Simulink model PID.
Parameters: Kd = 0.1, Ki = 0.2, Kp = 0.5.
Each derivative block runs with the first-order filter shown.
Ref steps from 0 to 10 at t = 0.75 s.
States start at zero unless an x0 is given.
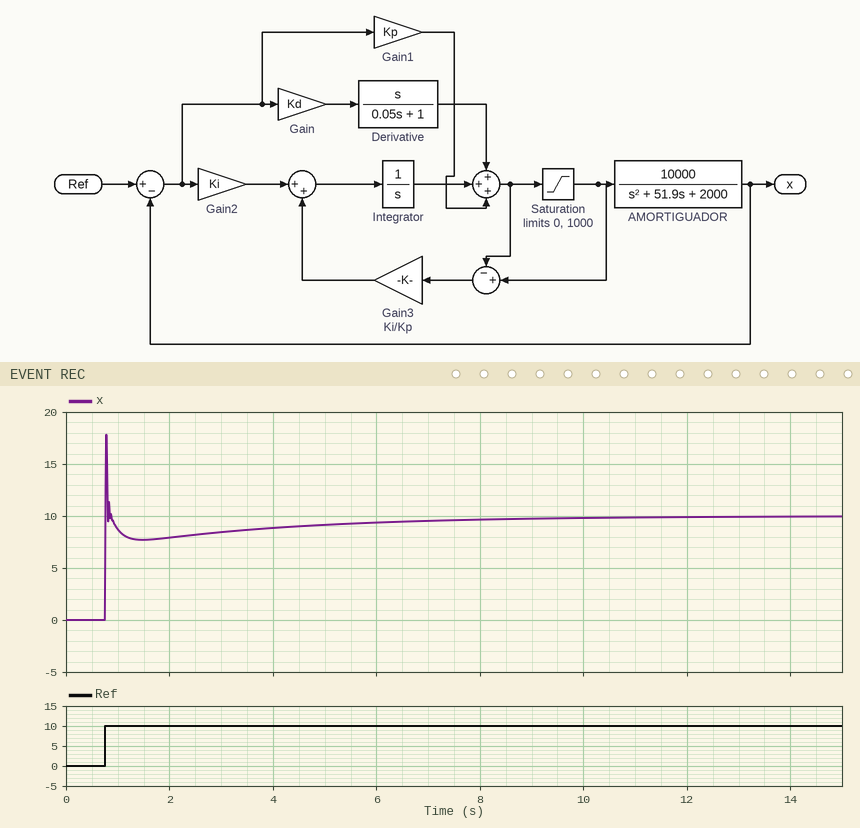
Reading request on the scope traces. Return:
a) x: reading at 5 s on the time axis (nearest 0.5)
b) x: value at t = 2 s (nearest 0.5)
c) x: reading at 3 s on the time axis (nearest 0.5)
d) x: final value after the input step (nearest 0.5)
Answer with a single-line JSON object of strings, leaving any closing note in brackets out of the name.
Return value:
{"x: reading at 5 s on the time axis": "9.0", "x: value at t = 2 s": "8.0", "x: reading at 3 s on the time axis": "8.5", "x: final value after the input step": "10.0"}
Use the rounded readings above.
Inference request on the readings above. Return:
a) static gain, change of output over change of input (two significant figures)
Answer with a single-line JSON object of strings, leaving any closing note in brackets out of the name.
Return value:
{"static gain, change of output over change of input": "1.0"}
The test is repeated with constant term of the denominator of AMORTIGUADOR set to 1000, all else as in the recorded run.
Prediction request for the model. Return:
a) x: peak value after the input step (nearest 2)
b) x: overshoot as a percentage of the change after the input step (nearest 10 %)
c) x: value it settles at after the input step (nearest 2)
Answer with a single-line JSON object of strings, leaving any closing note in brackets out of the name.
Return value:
{"x: peak value after the input step": "20", "x: overshoot as a percentage of the change after the input step": "110 %", "x: value it settles at after the input step": "10"}
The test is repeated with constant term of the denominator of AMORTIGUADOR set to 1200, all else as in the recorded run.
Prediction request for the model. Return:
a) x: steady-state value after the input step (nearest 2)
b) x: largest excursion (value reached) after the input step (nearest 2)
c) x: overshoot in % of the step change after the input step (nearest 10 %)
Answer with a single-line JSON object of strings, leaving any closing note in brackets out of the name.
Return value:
{"x: steady-state value after the input step": "10", "x: largest excursion (value reached) after the input step": "20", "x: overshoot in % of the step change after the input step": "100 %"}
